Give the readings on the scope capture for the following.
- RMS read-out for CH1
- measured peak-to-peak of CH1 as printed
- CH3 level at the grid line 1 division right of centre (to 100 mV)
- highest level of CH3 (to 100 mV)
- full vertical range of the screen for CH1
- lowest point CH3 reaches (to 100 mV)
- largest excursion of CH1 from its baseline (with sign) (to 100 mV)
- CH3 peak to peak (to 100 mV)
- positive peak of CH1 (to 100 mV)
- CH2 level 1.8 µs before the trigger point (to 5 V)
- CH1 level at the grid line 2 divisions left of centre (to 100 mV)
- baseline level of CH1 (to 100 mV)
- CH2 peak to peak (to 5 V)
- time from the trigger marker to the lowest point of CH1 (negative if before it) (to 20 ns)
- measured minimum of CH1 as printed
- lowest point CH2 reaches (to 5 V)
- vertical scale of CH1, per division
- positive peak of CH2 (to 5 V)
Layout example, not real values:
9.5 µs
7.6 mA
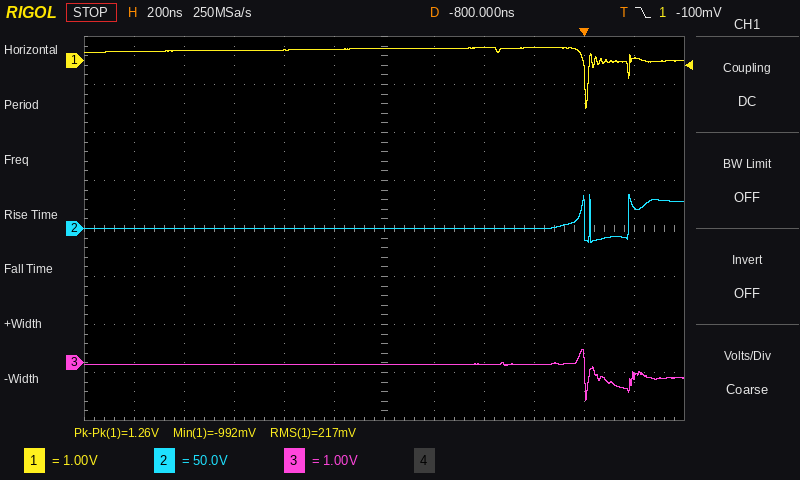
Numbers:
217 mV
1.26 V
0.0 V
300 mV
8 V
-800 mV
-1.2 V
1.1 V
300 mV
0 V
200 mV
200 mV
50 V
0 ns
-992 mV
-15 V
1 V
35 V
